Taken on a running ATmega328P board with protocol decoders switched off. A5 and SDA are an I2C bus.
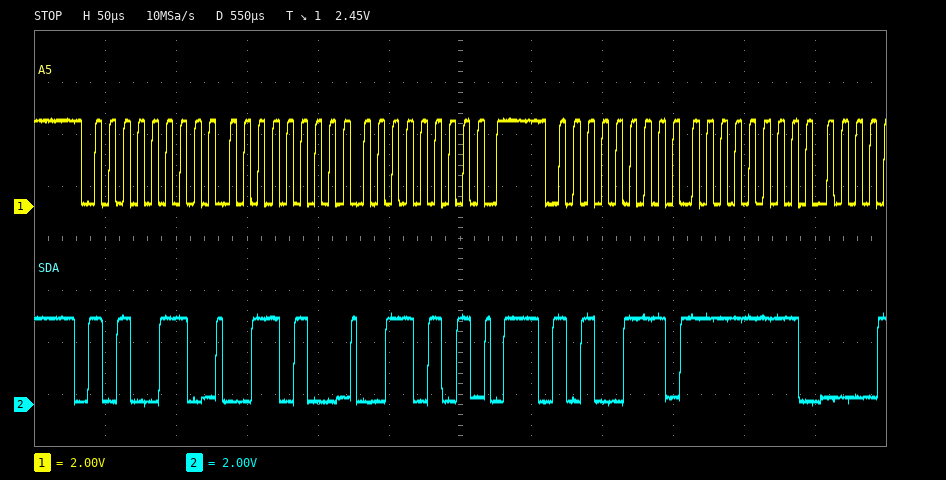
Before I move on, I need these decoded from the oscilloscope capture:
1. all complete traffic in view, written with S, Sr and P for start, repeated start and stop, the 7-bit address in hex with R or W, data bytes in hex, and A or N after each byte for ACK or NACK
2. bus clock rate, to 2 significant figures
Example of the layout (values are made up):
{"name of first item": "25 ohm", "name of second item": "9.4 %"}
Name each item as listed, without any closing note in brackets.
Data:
{"all complete traffic in view, written with S, Sr and P for start, repeated start and stop, the 7-bit address in hex with R or W, data bytes in hex, and A or N after each byte for ACK or NACK": "S 53W A 34 A 35 A P S 53R A FF A", "bus clock rate, to 2 significant figures": "100 kHz"}
